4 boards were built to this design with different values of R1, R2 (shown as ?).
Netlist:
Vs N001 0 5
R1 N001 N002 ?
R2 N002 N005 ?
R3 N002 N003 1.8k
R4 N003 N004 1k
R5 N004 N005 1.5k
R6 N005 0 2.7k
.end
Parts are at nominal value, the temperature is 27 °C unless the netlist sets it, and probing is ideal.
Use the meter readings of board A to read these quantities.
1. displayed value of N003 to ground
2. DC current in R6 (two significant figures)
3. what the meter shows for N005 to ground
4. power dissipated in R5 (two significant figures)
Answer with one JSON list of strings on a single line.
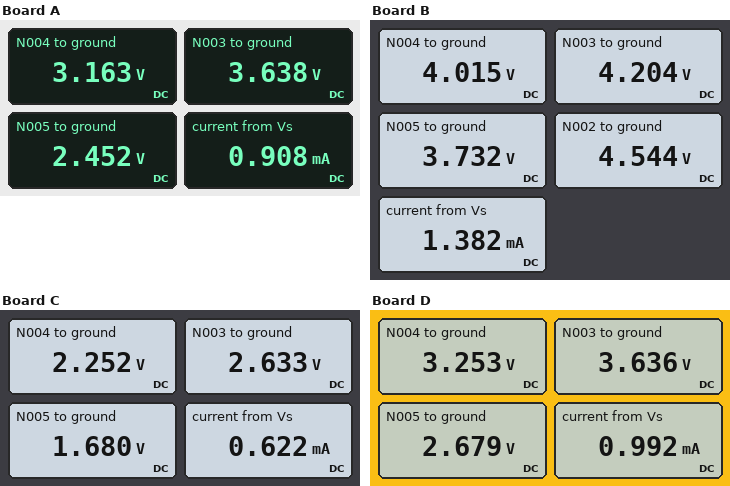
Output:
["3.638 V", "910 µA", "2.452 V", "340 µW"]
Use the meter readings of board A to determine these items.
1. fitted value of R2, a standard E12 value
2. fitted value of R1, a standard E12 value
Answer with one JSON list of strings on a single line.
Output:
["4.7 kΩ", "560 Ω"]
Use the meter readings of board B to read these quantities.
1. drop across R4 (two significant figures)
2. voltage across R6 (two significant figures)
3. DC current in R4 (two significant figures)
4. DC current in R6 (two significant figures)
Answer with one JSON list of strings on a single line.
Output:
["190 mV", "3.7 V", "190 µA", "1.4 mA"]
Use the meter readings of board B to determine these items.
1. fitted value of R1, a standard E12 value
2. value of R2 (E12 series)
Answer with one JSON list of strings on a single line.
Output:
["330 Ω", "680 Ω"]
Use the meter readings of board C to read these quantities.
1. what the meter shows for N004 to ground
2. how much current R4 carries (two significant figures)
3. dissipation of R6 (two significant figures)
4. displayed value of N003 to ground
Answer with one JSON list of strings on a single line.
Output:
["2.252 V", "380 µA", "1.0 mW", "2.633 V"]
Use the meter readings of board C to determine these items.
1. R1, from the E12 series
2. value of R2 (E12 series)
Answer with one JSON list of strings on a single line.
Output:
["2.7 kΩ", "6.8 kΩ"]
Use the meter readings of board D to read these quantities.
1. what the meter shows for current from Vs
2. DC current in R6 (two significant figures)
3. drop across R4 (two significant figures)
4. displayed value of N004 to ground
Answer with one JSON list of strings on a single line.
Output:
["0.992 mA", "990 µA", "380 mV", "3.253 V"]
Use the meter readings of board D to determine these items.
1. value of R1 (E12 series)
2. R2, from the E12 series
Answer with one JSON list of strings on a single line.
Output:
["680 Ω", "2.7 kΩ"]
